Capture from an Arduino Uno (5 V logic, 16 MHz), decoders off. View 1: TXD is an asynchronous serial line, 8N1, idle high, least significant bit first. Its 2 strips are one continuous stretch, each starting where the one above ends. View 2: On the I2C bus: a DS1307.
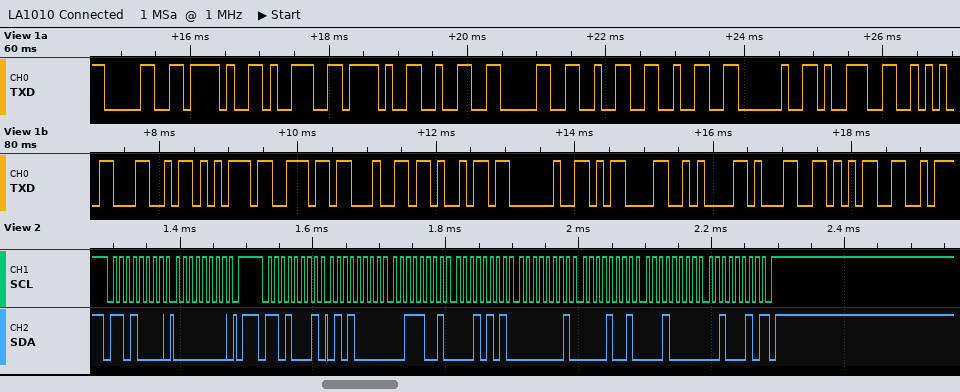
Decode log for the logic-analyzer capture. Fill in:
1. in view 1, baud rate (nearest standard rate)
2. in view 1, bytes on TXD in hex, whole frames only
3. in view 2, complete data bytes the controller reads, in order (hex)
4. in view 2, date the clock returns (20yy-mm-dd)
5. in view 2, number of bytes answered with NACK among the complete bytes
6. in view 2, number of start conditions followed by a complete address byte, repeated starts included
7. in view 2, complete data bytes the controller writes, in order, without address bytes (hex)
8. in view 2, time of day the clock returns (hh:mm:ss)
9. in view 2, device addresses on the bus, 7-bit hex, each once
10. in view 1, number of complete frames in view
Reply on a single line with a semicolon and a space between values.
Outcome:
9600 baud; 30 2F 39 2F 32 30 32 32 20 39 2A 4C 75 6E 64 69 20 0D 0A 31 35; 50 39 15 01 09 10 22; 2022-10-09; 1; 2; 00; 15:39:50; 0x68; 21
